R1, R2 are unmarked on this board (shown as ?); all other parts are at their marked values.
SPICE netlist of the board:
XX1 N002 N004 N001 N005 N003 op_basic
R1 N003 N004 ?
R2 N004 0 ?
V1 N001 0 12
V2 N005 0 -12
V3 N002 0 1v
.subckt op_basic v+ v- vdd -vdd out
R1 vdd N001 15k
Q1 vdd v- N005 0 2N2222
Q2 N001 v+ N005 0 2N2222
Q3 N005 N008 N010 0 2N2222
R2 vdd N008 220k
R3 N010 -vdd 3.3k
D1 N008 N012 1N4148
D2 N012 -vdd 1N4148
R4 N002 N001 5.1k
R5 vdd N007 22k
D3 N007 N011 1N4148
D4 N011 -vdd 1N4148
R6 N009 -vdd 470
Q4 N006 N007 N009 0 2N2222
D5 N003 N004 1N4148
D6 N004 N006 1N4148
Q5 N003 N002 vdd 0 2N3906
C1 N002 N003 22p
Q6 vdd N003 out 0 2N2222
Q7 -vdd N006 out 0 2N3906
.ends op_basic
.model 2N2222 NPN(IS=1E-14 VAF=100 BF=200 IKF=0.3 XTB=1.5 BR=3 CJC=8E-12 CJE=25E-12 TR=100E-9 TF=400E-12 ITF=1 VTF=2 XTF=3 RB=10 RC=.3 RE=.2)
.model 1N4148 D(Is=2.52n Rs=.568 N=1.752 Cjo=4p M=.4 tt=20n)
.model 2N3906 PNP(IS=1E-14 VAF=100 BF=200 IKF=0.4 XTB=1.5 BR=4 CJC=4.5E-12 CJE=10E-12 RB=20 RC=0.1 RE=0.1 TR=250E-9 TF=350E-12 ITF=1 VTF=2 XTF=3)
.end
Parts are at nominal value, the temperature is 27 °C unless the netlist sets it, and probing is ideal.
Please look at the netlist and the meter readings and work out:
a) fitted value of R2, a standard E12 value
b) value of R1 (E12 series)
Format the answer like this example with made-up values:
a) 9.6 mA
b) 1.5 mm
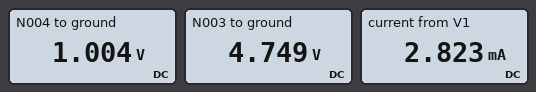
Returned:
a) 2.2 kΩ
b) 8.2 kΩ
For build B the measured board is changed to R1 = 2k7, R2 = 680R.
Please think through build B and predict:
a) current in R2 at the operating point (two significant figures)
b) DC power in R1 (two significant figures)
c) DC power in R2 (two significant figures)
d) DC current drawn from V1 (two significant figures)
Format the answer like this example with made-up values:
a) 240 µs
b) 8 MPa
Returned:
a) 1.5 mA
b) 5.9 mW
c) 1.5 mW
d) 3.8 mA
